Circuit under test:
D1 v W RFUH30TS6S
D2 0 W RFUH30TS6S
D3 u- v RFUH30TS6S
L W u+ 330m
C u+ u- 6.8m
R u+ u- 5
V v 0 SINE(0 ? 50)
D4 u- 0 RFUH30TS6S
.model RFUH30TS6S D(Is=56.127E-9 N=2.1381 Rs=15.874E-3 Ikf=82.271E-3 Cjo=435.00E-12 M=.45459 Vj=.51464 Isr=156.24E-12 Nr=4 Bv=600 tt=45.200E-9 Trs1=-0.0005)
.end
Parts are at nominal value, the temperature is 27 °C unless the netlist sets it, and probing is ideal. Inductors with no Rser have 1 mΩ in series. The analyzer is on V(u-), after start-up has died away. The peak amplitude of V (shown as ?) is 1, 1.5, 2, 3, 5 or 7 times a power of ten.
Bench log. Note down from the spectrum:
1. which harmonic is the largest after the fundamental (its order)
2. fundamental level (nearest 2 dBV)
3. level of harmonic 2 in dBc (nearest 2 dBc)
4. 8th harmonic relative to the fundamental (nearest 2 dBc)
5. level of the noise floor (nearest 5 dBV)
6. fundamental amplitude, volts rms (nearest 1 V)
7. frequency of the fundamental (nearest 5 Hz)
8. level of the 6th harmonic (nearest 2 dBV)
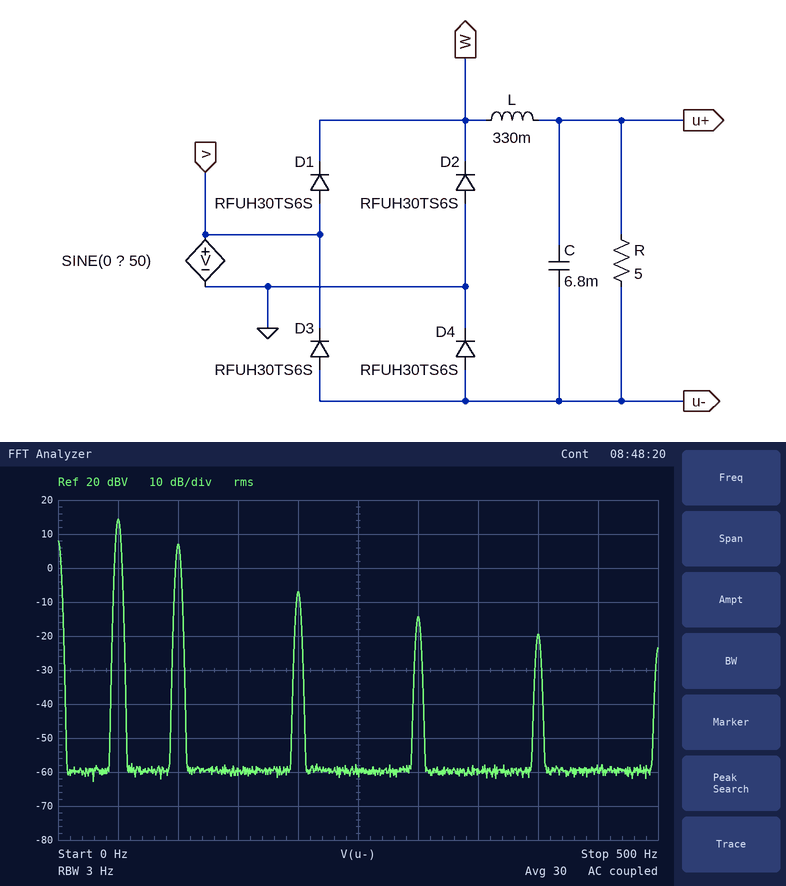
2
14 dBV
-8 dBc
-34 dBc
-60 dBV
5 V
50 Hz
-14 dBV
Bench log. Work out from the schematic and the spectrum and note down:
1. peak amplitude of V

15 V
